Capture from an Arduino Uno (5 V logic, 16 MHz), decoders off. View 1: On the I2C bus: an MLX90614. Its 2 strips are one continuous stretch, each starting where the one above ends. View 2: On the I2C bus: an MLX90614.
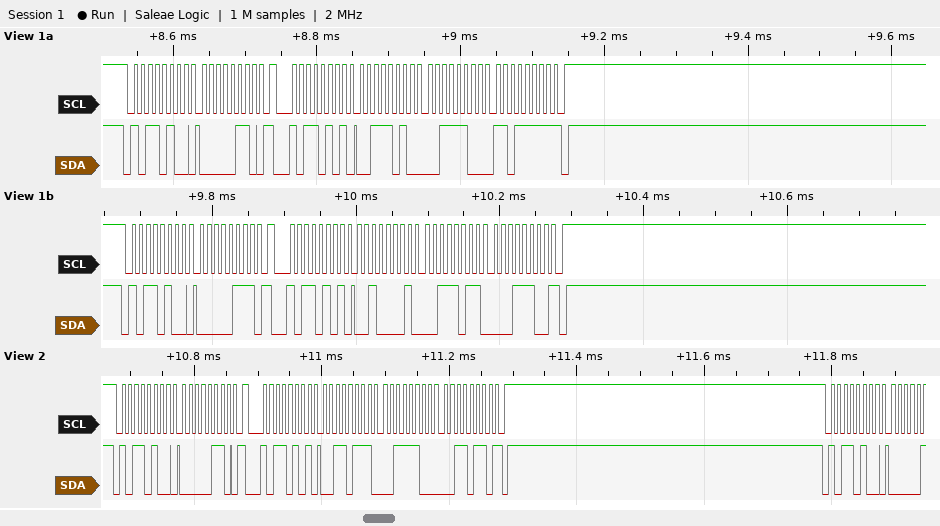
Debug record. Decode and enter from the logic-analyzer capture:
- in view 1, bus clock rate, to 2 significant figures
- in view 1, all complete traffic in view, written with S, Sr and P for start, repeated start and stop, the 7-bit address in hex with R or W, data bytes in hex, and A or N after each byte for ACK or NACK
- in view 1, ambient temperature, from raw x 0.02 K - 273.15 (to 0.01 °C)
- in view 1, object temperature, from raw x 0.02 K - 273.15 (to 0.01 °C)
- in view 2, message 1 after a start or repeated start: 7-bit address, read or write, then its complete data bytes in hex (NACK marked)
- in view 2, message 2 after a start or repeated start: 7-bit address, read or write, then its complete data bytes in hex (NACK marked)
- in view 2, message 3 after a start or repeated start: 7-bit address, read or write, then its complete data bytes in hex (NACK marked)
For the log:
100 kHz
S 5AW A 06 A Sr 5AR A 3A A 3C A DF N P S 5AW A 07 A Sr 5AR A 21 A 3B A 1C N P
35.21 °C
29.59 °C
0x5A write: 06
0x5A read: 37 3C 36 NACK
0x5A write
